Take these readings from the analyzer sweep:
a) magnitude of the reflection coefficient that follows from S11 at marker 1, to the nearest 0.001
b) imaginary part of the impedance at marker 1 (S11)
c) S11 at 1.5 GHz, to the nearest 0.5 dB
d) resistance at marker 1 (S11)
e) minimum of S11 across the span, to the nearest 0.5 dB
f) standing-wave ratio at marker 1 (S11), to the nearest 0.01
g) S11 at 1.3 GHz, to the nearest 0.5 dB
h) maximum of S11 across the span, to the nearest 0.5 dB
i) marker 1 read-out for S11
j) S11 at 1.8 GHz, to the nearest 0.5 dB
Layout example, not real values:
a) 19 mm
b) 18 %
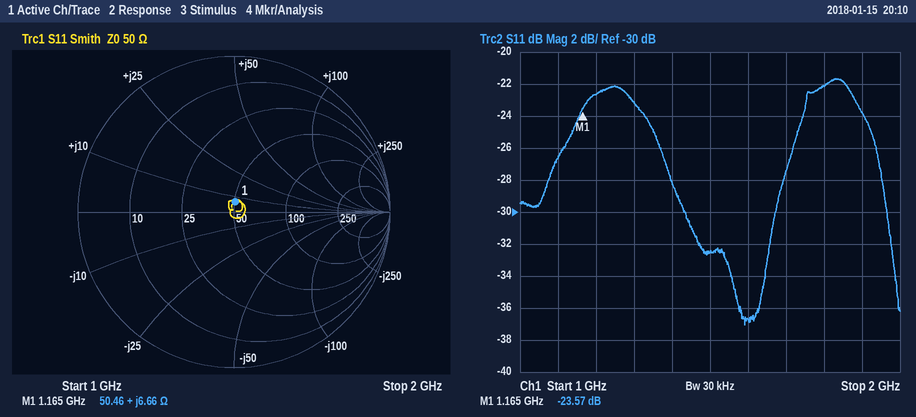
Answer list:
a) 0.066
b) +6.66 Ω
c) -32.5 dB
d) 50.46 Ω
e) -37.0 dB
f) 1.14
g) -23.0 dB
h) -21.5 dB
i) -23.57 dB
j) -22.0 dB
